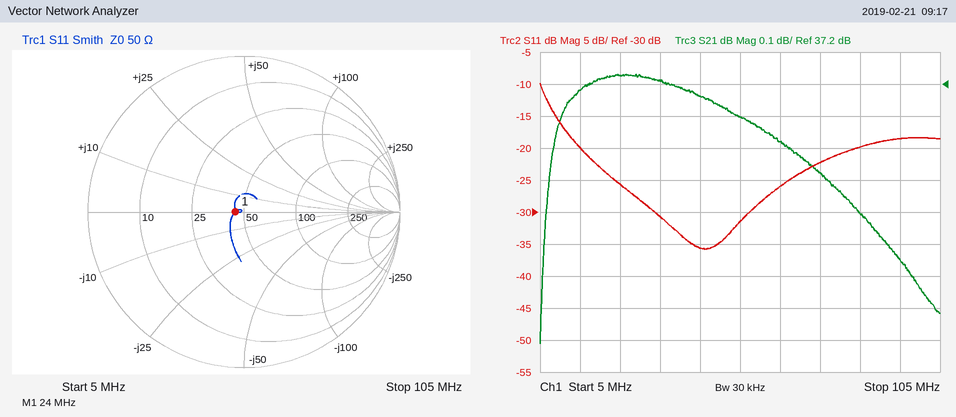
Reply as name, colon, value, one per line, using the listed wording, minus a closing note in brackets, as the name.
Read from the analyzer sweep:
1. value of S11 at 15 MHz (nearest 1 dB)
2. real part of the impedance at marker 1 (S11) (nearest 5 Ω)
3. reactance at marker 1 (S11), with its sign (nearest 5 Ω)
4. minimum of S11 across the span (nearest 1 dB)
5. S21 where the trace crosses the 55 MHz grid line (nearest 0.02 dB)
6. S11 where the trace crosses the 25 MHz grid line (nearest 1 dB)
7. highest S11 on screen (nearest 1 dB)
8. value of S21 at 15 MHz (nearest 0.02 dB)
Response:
value of S11 at 15 MHz: -20 dB
real part of the impedance at marker 1 (S11): 45 Ω
reactance at marker 1 (S11), with its sign: 0 Ω
minimum of S11 across the span: -36 dB
S21 where the trace crosses the 55 MHz grid line: 37.10 dB
S11 where the trace crosses the 25 MHz grid line: -26 dB
highest S11 on screen: -10 dB
value of S21 at 15 MHz: 37.18 dB
